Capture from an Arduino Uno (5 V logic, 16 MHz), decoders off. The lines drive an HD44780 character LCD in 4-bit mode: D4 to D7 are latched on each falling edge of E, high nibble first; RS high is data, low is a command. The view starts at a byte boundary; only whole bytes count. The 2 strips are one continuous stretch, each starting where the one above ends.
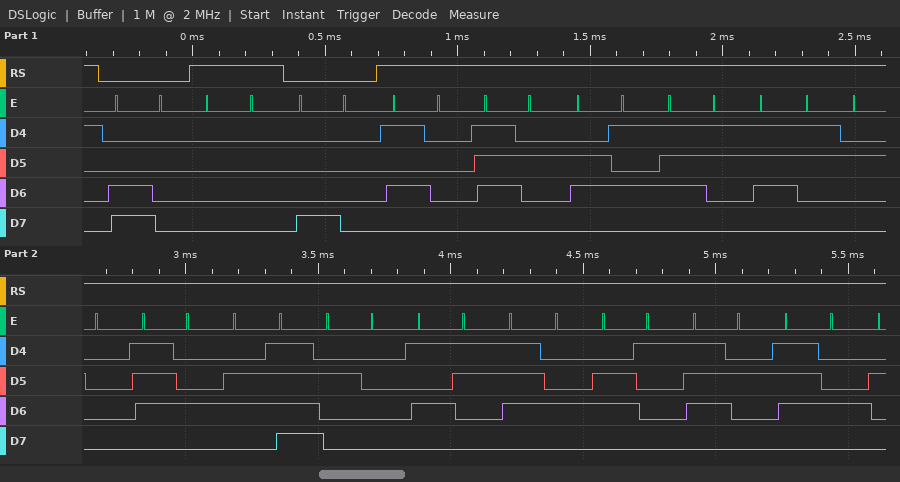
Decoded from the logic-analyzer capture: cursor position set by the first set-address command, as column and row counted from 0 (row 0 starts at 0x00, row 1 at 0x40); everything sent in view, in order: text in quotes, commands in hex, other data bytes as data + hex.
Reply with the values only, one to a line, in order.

column 0, row 1
0xC0 data 00 0x80 "Press to Start"
